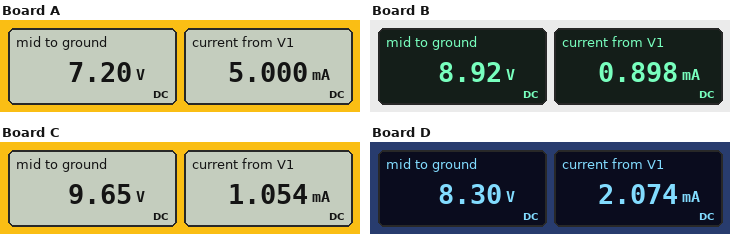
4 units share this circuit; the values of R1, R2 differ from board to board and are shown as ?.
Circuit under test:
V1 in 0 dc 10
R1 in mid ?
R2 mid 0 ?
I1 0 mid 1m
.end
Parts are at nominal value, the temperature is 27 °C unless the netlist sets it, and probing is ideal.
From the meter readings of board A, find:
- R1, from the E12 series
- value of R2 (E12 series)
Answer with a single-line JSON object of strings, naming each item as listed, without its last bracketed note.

{"R1, from the E12 series": "560 Ω", "value of R2": "1.2 kΩ"}
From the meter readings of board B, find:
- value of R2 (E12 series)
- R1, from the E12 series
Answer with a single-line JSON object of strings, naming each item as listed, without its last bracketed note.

{"value of R2": "4.7 kΩ", "R1, from the E12 series": "1.2 kΩ"}
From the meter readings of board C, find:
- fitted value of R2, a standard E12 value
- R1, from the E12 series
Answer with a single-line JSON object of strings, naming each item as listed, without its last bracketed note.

{"fitted value of R2, a standard E12 value": "4.7 kΩ", "R1, from the E12 series": "330 Ω"}
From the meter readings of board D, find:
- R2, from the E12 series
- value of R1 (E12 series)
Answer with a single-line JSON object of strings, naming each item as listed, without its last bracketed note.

{"R2, from the E12 series": "2.7 kΩ", "value of R1": "820 Ω"}
